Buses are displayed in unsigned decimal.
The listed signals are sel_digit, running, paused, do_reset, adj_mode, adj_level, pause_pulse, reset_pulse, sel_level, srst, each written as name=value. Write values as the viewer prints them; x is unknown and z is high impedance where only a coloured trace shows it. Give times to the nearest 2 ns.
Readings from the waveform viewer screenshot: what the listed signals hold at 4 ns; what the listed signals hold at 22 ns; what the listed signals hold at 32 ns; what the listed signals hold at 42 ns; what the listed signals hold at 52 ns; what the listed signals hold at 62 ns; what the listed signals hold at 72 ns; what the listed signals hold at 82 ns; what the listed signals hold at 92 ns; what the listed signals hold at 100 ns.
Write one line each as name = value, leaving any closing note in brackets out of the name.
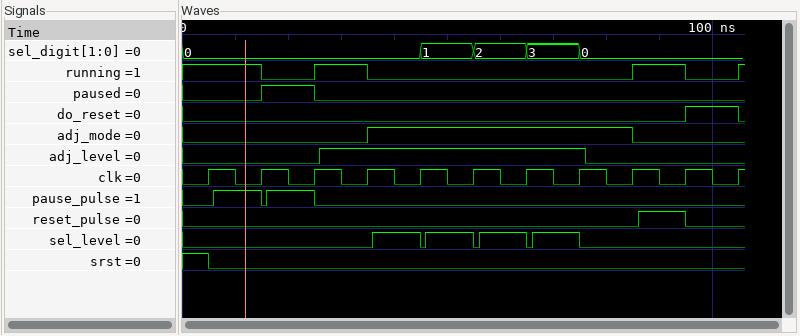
what the listed signals hold at 4 ns = sel_digit=0, running=1, paused=0, do_reset=0, adj_mode=0, adj_level=0, pause_pulse=0, reset_pulse=0, sel_level=0, srst=1
what the listed signals hold at 22 ns = sel_digit=0, running=0, paused=1, do_reset=0, adj_mode=0, adj_level=0, pause_pulse=1, reset_pulse=0, sel_level=0, srst=0
what the listed signals hold at 32 ns = sel_digit=0, running=1, paused=0, do_reset=0, adj_mode=0, adj_level=1, pause_pulse=0, reset_pulse=0, sel_level=0, srst=0
what the listed signals hold at 42 ns = sel_digit=0, running=0, paused=0, do_reset=0, adj_mode=1, adj_level=1, pause_pulse=0, reset_pulse=0, sel_level=1, srst=0
what the listed signals hold at 52 ns = sel_digit=1, running=0, paused=0, do_reset=0, adj_mode=1, adj_level=1, pause_pulse=0, reset_pulse=0, sel_level=1, srst=0
what the listed signals hold at 62 ns = sel_digit=2, running=0, paused=0, do_reset=0, adj_mode=1, adj_level=1, pause_pulse=0, reset_pulse=0, sel_level=1, srst=0
what the listed signals hold at 72 ns = sel_digit=3, running=0, paused=0, do_reset=0, adj_mode=1, adj_level=1, pause_pulse=0, reset_pulse=0, sel_level=1, srst=0
what the listed signals hold at 82 ns = sel_digit=0, running=0, paused=0, do_reset=0, adj_mode=1, adj_level=0, pause_pulse=0, reset_pulse=0, sel_level=0, srst=0
what the listed signals hold at 92 ns = sel_digit=0, running=1, paused=0, do_reset=0, adj_mode=0, adj_level=0, pause_pulse=0, reset_pulse=1, sel_level=0, srst=0
what the listed signals hold at 100 ns = sel_digit=0, running=0, paused=0, do_reset=1, adj_mode=0, adj_level=0, pause_pulse=0, reset_pulse=0, sel_level=0, srst=0
